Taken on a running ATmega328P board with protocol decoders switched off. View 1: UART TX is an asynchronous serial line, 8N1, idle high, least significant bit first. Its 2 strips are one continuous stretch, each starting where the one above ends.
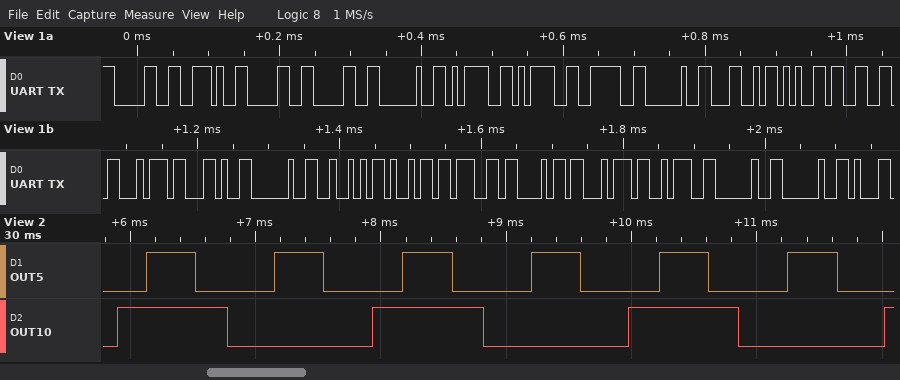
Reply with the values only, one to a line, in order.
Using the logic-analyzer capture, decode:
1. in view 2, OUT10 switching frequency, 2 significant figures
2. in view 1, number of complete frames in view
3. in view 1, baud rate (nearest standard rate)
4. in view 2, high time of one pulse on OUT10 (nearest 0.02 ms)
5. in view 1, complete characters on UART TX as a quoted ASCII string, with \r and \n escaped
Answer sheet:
490 Hz
23
115200 baud
0.88 ms
"0.00 ==> Left, Right:  "
